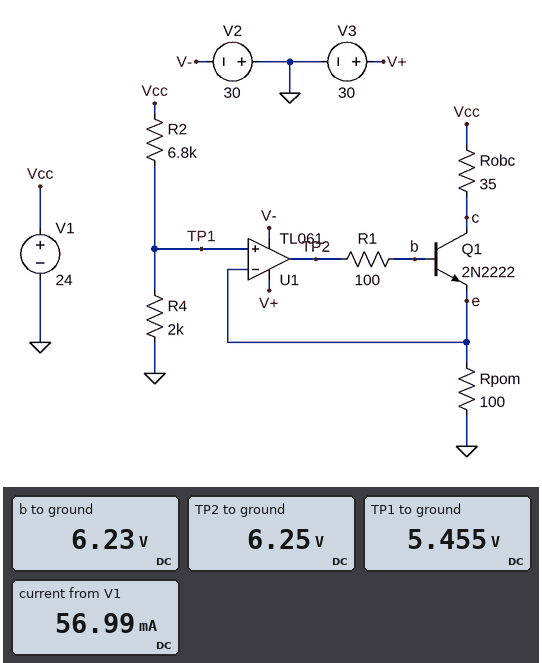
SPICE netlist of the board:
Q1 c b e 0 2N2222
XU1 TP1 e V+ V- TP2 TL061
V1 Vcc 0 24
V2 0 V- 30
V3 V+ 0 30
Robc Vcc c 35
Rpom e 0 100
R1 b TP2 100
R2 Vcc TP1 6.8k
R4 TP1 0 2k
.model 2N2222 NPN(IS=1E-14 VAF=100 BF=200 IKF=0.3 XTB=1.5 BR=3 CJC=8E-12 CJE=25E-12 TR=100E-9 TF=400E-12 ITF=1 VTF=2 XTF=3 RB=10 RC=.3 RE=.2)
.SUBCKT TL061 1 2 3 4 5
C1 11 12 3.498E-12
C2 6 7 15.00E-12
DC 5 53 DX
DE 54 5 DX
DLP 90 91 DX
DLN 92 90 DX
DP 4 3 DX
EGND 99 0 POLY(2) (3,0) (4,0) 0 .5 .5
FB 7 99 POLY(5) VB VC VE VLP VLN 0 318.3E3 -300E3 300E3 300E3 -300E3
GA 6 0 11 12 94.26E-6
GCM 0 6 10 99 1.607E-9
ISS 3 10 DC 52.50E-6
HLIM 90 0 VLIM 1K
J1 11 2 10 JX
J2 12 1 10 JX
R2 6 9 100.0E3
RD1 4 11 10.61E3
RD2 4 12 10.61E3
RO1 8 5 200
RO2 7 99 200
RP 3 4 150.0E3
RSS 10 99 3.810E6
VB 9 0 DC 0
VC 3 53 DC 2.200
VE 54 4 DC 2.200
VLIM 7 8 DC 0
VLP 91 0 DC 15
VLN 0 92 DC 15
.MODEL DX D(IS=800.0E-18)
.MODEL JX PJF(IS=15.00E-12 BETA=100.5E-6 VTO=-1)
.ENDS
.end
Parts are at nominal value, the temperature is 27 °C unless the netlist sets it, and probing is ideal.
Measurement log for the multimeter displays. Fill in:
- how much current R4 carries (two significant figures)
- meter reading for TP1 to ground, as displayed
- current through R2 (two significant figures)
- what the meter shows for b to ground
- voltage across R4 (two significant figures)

2.7 mA
5.455 V
2.7 mA
6.23 V
5.5 V
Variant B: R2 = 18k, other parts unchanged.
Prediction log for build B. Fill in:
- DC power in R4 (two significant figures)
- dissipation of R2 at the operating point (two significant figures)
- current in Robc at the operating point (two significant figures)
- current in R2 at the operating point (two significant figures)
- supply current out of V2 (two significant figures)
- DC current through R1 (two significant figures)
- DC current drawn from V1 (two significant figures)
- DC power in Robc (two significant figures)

2.9 mW
26 mW
24 mA
1.2 mA
450 µA
110 µA
25 mA
20 mW
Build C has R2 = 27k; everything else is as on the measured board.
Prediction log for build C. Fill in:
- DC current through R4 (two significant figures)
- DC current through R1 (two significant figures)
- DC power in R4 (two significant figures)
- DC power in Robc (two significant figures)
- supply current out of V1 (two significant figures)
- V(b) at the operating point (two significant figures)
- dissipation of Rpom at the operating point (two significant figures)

830 µA
71 µA
1.4 mW
9.5 mW
17 mA
2.4 V
27 mW
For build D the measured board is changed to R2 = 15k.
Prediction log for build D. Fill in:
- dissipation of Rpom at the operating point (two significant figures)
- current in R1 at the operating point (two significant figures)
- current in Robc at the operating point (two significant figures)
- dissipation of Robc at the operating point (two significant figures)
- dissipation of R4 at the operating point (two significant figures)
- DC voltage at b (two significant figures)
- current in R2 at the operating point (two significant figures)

80 mW
130 µA
28 mA
28 mW
4.0 mW
3.6 V
1.4 mA
